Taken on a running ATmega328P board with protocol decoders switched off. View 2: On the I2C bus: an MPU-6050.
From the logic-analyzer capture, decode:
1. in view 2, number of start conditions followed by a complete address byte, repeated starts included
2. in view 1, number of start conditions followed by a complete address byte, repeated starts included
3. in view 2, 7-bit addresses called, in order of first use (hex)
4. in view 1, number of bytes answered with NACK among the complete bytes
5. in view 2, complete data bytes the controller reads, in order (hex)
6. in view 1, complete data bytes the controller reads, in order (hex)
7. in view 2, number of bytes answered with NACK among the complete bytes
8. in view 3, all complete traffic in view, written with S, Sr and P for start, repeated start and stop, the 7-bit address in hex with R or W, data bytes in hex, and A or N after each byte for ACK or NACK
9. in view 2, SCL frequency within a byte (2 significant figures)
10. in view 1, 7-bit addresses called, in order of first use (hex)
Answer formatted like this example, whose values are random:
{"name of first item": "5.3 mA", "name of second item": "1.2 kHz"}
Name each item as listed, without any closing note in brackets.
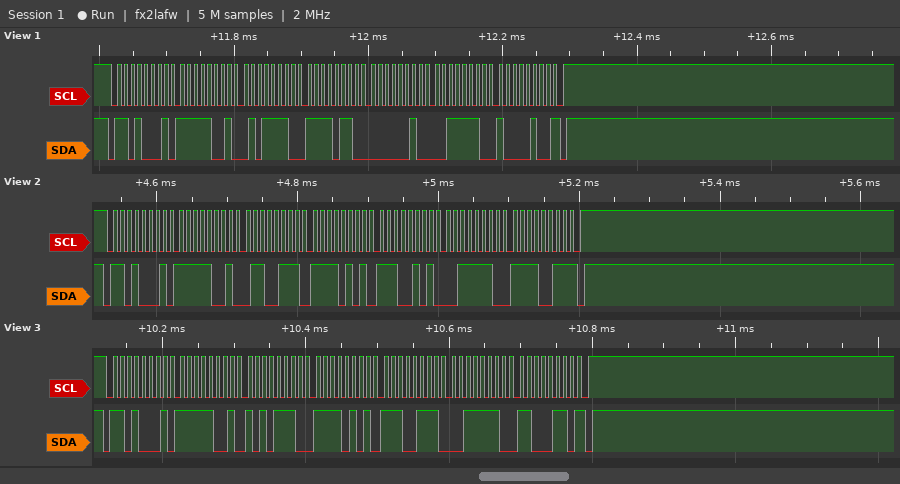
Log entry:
{"in view 2, number of start conditions followed by a complete address byte, repeated starts included": "1", "in view 1, number of start conditions followed by a complete address byte, repeated starts included": "1", "in view 2, 7-bit addresses called, in order of first use": "0x68", "in view 1, number of bytes answered with NACK among the complete bytes": "1", "in view 2, complete data bytes the controller reads, in order": "F9 67 F5 E5 3E F3", "in view 1, complete data bytes the controller reads, in order": "F9 5E F6 02 3E 84", "in view 2, number of bytes answered with NACK among the complete bytes": "1", "in view 3, all complete traffic in view, written with S, Sr and P for start, repeated start and stop, the 7-bit address in hex with R or W, data bytes in hex, and A or N after each byte for ACK or NACK": "S 68R A F9 A AE A F5 A E7 A 3E A C6 N P", "in view 2, SCL frequency within a byte": "100 kHz", "in view 1, 7-bit addresses called, in order of first use": "0x68"}
